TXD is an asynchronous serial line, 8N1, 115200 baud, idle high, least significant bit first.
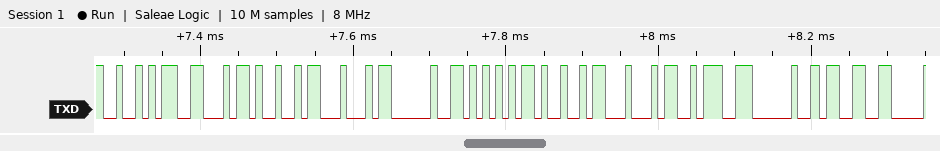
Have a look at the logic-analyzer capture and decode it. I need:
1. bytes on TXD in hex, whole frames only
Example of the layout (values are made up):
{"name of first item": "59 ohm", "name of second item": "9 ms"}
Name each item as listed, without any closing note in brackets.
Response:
{"bytes on TXD in hex, whole frames only": "0x52 0x46 0x49 0x44 0x20 0x55 0x49 0x44 0x3A 0x20 0x33"}
